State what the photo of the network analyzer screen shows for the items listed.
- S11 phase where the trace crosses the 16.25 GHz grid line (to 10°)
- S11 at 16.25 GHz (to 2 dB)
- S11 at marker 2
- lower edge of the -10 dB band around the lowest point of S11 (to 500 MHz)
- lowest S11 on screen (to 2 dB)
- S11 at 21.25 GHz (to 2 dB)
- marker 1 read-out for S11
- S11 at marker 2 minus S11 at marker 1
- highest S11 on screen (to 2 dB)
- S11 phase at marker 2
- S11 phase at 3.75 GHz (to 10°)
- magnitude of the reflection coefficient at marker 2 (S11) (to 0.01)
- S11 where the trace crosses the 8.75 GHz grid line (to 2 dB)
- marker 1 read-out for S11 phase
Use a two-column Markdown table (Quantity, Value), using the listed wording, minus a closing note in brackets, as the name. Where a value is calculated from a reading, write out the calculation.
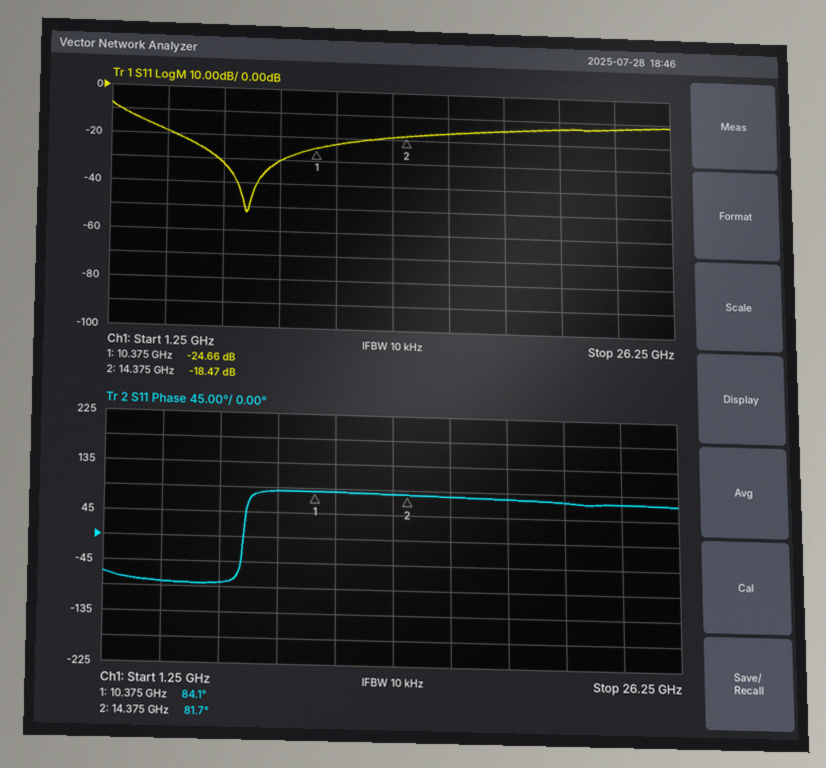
| Quantity | Value |
|---|---|
| S11 phase where the trace crosses the 16.25 GHz grid line | 80° |
| S11 at 16.25 GHz | -16 dB |
| S11 at marker 2 | -18.47 dB |
| lower edge of the -10 dB band around the lowest point of S11 | 1.5 GHz |
| lowest S11 on screen | -52 dB |
| S11 at 21.25 GHz | -14 dB |
| marker 1 read-out for S11 | -24.66 dB |
| S11 at marker 2 minus S11 at marker 1 | -18.47 − (-24.66) = 6.19 dB |
| highest S11 on screen | -8 dB |
| S11 phase at marker 2 | 81.7° |
| S11 phase at 3.75 GHz | -80° |
| magnitude of the reflection coefficient at marker 2 (S11) | 10^(-18.47/20) ≈ 0.12 |
| S11 where the trace crosses the 8.75 GHz grid line | -30 dB |
| marker 1 read-out for S11 phase | 84.1° |
